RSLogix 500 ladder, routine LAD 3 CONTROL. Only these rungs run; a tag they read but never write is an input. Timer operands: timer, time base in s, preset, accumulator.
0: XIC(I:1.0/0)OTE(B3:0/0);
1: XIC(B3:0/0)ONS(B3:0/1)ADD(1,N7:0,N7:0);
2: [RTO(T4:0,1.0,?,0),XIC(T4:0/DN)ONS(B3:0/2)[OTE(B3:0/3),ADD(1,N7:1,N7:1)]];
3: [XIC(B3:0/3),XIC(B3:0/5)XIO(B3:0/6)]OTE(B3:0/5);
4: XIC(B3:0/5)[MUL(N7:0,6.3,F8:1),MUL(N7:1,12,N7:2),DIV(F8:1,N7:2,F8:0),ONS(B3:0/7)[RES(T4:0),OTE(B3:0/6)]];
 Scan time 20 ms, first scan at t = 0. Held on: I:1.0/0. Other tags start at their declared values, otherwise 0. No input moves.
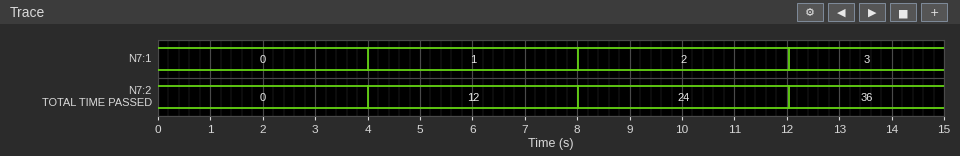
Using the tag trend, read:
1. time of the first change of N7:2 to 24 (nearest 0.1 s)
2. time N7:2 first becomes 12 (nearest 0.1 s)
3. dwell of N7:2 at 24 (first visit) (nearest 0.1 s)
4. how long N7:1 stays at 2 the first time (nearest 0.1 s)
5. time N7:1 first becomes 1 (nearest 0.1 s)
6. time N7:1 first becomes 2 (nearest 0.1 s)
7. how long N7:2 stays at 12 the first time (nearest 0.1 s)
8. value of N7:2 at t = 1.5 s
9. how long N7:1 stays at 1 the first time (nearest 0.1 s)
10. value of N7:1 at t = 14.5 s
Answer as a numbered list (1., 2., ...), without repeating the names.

1. 8.0 s
2. 4.0 s
3. 4.0 s
4. 4.0 s
5. 4.0 s
6. 8.0 s
7. 4.0 s
8. 0
9. 4.0 s
10. 3
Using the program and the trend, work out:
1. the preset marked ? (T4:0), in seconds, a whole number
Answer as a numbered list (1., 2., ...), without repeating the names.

1. 4 s
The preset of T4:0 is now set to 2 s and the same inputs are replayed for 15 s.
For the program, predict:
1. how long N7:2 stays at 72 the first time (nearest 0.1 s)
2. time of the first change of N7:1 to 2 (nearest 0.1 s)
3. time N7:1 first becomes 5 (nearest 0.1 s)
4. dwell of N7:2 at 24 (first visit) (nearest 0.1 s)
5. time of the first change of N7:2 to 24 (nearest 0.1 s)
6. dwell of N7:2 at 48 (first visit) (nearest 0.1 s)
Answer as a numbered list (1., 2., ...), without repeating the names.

1. 2.0 s
2. 4.0 s
3. 10.1 s
4. 2.0 s
5. 4.0 s
6. 2.0 s
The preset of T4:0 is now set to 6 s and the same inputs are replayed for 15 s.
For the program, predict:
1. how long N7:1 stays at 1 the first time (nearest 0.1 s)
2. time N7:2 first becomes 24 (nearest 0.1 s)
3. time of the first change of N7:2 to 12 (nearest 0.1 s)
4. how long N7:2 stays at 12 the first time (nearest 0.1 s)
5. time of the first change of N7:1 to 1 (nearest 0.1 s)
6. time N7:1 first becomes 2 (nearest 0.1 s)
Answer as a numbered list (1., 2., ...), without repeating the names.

1. 6.0 s
2. 12.0 s
3. 6.0 s
4. 6.0 s
5. 6.0 s
6. 12.0 s
